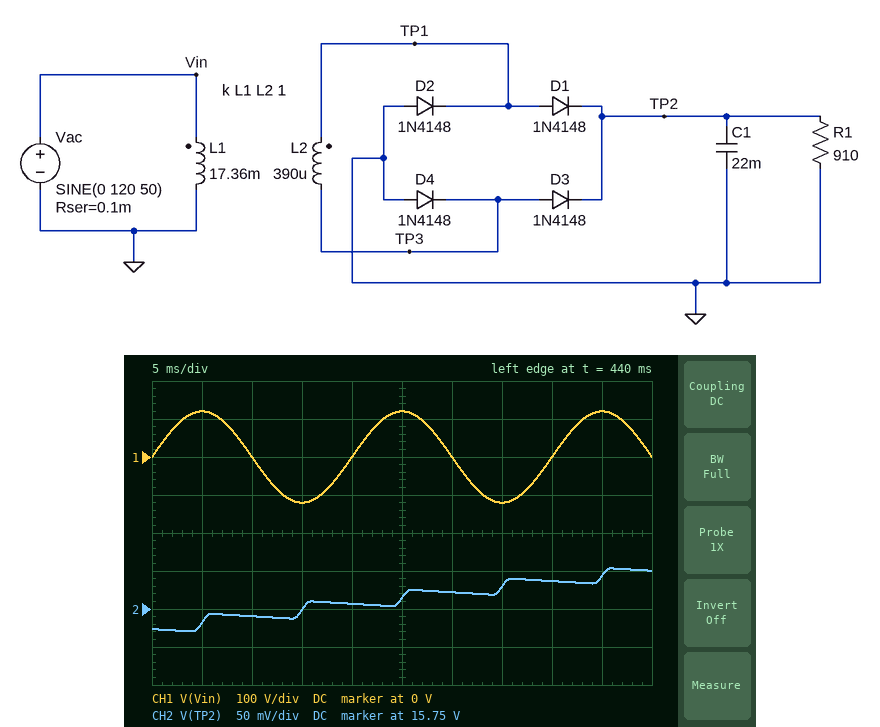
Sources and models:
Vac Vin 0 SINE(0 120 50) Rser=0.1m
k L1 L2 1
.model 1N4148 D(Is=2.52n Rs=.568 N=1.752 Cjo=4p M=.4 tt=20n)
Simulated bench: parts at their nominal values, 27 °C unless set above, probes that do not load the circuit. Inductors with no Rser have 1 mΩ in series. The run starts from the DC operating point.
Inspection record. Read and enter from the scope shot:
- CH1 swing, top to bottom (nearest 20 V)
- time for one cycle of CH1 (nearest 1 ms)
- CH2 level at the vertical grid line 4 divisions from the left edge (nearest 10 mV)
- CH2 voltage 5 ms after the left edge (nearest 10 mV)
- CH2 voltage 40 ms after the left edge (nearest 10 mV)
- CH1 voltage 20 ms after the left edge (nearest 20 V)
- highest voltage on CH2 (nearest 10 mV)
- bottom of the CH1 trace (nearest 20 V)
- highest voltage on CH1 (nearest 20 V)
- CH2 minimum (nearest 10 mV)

240 V
20 ms
15.76 V
15.73 V
15.79 V
0 V
15.80 V
-120 V
120 V
15.72 V
